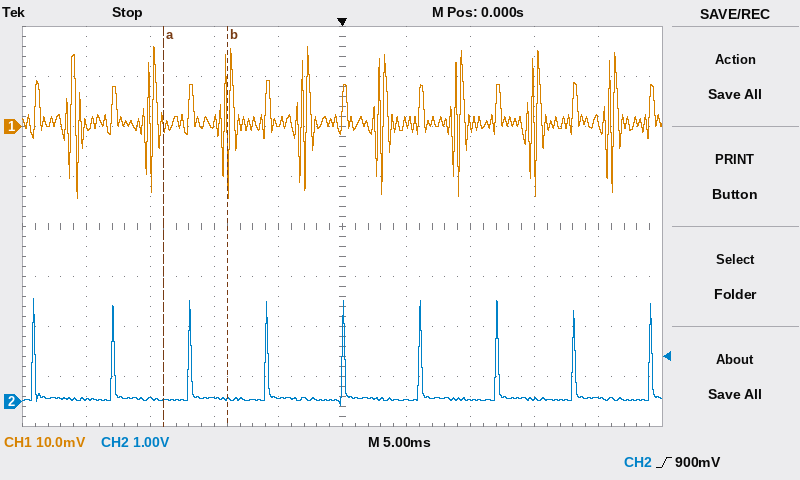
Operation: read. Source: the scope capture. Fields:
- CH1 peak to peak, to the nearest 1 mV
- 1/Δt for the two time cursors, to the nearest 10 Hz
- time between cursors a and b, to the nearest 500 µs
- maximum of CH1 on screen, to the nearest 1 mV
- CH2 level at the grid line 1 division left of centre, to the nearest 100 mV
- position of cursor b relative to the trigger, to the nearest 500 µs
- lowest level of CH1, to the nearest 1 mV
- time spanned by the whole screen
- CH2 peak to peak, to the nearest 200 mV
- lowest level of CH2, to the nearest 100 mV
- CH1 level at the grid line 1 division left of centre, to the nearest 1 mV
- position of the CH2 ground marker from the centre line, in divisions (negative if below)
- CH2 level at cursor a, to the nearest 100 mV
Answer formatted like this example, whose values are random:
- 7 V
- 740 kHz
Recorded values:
- 30 mV
- 200 Hz
- 5.0 ms
- 16 mV
- 100 mV
- -9.0 ms
- -14 mV
- 50 ms
- 2.2 V
- -100 mV
- 1 mV
- -3.5 div
- 0.0 V
